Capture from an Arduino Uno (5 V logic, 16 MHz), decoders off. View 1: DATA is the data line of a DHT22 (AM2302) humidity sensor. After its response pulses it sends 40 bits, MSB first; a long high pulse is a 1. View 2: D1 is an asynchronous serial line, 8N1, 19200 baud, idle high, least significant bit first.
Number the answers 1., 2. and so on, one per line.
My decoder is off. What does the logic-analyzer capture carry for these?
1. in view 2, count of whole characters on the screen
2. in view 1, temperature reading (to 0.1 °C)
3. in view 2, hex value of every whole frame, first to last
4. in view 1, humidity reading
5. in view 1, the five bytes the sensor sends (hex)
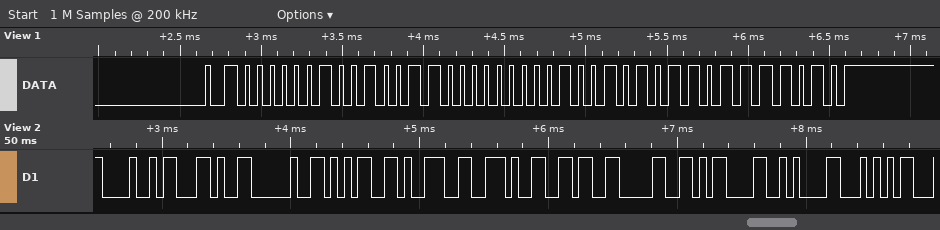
1. 11
2. 29.9 °C
3. 48 2C 20 35 39 2E 36 30 0D 0A 54
4. 58.8 %
5. 02 4C 01 2B 7A
